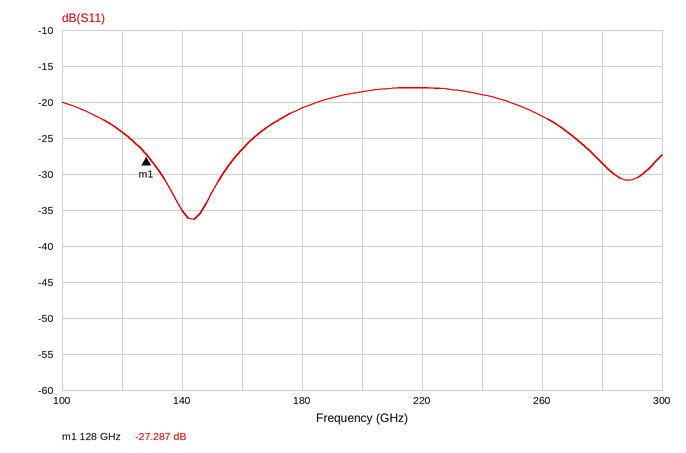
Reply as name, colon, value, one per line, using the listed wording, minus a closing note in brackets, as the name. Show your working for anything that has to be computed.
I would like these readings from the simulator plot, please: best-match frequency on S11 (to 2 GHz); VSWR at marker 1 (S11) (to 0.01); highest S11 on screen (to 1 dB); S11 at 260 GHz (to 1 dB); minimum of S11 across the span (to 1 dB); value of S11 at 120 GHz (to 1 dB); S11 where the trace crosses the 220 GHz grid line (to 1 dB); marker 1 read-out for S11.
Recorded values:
best-match frequency on S11: 144 GHz
VSWR at marker 1 (S11): (1 + 0.0432)/(1 − 0.0432) ≈ 1.09
highest S11 on screen: -18 dB
S11 at 260 GHz: -22 dB
minimum of S11 across the span: -36 dB
value of S11 at 120 GHz: -24 dB
S11 where the trace crosses the 220 GHz grid line: -18 dB
marker 1 read-out for S11: -27.287 dB
